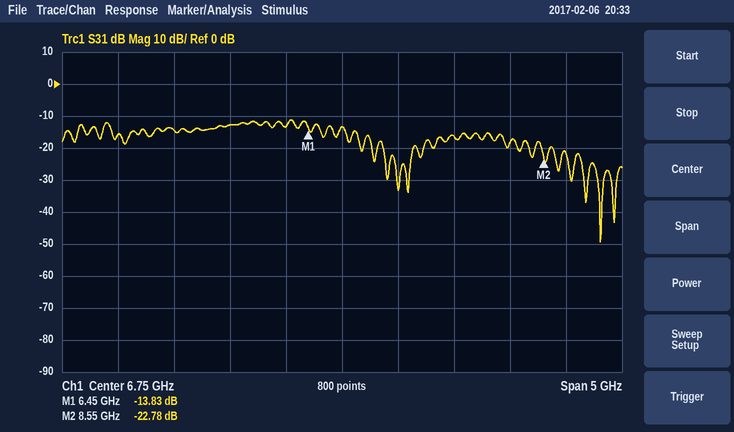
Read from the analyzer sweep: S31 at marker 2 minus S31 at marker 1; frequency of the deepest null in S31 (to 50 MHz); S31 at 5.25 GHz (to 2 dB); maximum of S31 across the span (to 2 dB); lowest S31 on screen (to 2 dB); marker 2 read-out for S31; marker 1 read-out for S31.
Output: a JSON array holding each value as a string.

["-8.95 dB", "9.05 GHz", "-14 dB", "-12 dB", "-50 dB", "-22.78 dB", "-13.83 dB"]
